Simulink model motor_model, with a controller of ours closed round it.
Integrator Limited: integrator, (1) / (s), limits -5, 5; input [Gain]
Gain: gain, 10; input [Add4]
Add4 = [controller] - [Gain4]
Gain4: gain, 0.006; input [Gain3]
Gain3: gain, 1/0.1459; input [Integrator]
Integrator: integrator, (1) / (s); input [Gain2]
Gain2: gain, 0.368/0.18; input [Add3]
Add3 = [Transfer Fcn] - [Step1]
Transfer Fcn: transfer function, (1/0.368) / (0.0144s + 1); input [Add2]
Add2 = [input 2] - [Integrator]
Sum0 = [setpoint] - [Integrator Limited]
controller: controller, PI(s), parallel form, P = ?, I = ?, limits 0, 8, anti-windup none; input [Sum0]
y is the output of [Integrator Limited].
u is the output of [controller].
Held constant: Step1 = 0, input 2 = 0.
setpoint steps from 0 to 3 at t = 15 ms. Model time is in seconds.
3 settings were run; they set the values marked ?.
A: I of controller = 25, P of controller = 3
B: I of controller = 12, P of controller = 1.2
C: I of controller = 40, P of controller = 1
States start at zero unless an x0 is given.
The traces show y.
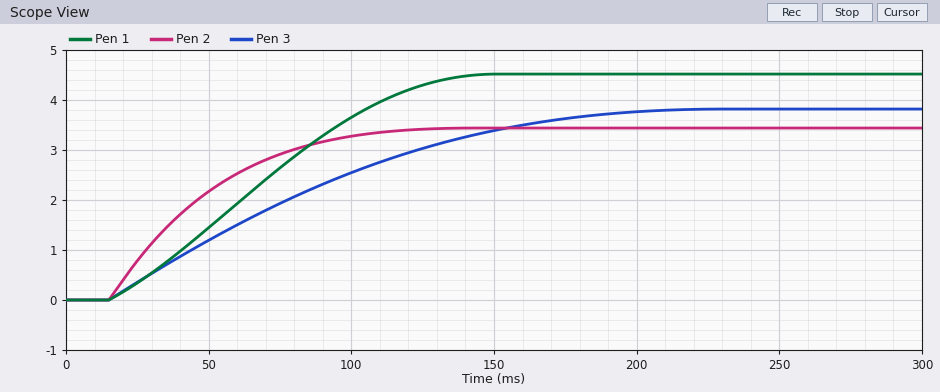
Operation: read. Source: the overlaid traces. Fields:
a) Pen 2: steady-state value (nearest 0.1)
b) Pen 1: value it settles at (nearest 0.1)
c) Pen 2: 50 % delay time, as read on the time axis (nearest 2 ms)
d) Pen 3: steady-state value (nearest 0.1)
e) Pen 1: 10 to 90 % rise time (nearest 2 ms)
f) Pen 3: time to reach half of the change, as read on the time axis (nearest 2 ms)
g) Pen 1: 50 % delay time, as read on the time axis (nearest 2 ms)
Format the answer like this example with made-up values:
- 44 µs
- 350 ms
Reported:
- 3.4
- 4.5
- 40 ms
- 3.8
- 86 ms
- 74 ms
- 66 ms
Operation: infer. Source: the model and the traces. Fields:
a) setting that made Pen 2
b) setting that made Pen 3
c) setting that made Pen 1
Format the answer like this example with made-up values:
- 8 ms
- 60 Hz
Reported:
- A
- B
- C
